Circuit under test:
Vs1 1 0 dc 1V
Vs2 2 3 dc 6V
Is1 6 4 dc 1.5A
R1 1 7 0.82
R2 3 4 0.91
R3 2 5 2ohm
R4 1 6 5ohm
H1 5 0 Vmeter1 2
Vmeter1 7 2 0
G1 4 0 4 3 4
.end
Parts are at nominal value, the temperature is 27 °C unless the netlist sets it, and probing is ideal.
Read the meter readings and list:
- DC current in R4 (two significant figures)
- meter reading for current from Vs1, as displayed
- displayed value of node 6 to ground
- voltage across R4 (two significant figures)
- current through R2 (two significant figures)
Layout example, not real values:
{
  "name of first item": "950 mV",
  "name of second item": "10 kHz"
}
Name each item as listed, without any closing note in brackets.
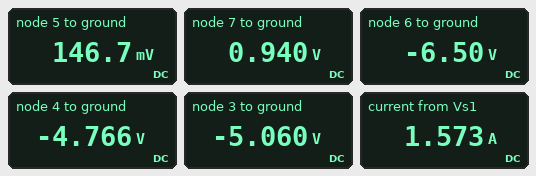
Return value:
{
  "DC current in R4": "1.5 A",
  "meter reading for current from Vs1, as displayed": "1.573 A",
  "displayed value of node 6 to ground": "-6.50 V",
  "voltage across R4": "7.5 V",
  "current through R2": "320 mA"
}
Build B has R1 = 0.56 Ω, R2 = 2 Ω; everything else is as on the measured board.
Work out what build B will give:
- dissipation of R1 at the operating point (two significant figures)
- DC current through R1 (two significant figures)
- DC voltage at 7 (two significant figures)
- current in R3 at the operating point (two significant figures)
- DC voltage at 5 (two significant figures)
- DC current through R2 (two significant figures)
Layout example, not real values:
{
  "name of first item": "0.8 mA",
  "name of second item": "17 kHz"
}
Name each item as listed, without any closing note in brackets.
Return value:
{
  "dissipation of R1 at the operating point": "12 mW",
  "DC current through R1": "150 mA",
  "DC voltage at 7": "920 mV",
  "current in R3 at the operating point": "310 mA",
  "DC voltage at 5": "290 mV",
  "DC current through R2": "170 mA"
}
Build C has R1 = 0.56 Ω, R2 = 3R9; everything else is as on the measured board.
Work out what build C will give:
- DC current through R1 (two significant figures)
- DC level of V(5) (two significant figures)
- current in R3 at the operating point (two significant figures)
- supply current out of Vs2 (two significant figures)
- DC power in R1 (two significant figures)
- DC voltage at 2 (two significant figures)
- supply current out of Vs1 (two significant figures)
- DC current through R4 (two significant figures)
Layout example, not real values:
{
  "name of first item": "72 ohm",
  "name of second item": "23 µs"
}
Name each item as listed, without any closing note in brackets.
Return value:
{
  "DC current through R1": "180 mA",
  "DC level of V(5)": "360 mV",
  "current in R3 at the operating point": "270 mA",
  "supply current out of Vs2": "90 mA",
  "DC power in R1": "18 mW",
  "DC voltage at 2": "900 mV",
  "supply current out of Vs1": "1.7 A",
  "DC current through R4": "1.5 A"
}
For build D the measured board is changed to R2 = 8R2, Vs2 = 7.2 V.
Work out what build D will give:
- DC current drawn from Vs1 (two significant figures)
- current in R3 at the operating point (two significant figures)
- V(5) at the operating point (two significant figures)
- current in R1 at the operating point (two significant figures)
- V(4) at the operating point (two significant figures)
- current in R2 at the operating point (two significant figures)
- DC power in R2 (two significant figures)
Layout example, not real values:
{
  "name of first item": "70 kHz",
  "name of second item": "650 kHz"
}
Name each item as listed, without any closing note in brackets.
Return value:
{
  "DC current drawn from Vs1": "1.7 A",
  "current in R3 at the operating point": "230 mA",
  "V(5) at the operating point": "380 mV",
  "current in R1 at the operating point": "190 mA",
  "V(4) at the operating point": "-6.0 V",
  "current in R2 at the operating point": "44 mA",
  "DC power in R2": "16 mW"
}
